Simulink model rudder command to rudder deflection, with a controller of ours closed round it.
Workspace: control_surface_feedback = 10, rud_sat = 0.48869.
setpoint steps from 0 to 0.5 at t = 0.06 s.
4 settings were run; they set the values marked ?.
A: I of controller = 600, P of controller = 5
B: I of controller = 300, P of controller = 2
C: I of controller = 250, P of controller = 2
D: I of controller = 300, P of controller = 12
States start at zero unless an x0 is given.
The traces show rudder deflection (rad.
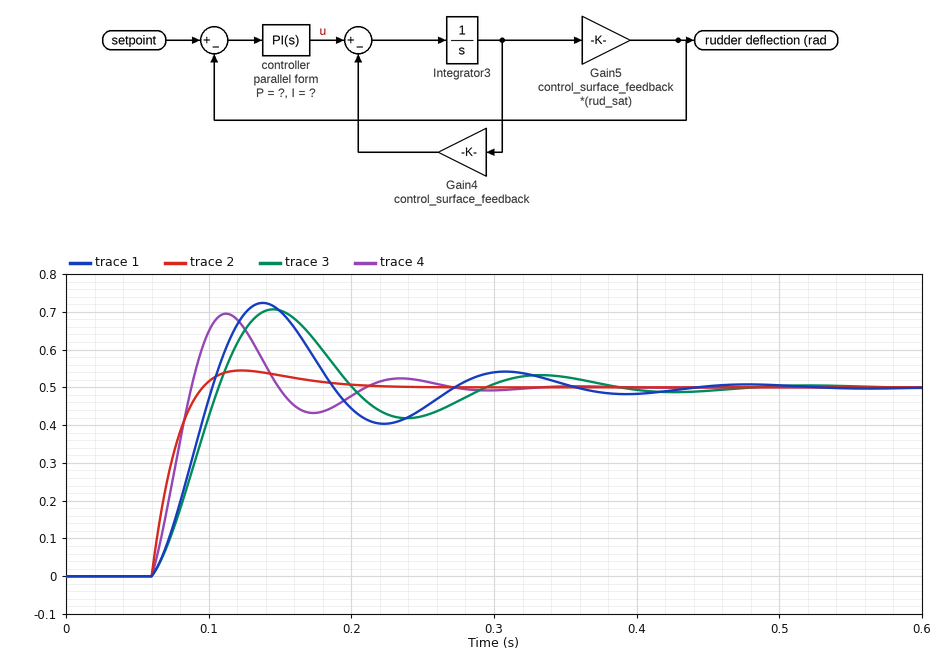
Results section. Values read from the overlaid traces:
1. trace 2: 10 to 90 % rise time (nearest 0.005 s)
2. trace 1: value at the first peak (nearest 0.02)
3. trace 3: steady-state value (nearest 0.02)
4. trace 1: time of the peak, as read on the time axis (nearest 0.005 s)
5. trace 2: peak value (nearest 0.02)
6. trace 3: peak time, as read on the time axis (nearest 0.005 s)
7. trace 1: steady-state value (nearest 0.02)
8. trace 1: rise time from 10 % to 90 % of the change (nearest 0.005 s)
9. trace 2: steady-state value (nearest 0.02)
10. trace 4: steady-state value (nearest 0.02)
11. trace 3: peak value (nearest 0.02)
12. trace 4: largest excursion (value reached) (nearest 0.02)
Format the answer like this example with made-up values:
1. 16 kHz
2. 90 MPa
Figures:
1. 0.025 s
2. 0.72
3. 0.50
4. 0.140 s
5. 0.54
6. 0.145 s
7. 0.50
8. 0.030 s
9. 0.50
10. 0.50
11. 0.70
12. 0.70
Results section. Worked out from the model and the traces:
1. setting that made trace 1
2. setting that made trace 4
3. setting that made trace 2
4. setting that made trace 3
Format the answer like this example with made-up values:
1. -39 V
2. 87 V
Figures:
1. B
2. A
3. D
4. C
